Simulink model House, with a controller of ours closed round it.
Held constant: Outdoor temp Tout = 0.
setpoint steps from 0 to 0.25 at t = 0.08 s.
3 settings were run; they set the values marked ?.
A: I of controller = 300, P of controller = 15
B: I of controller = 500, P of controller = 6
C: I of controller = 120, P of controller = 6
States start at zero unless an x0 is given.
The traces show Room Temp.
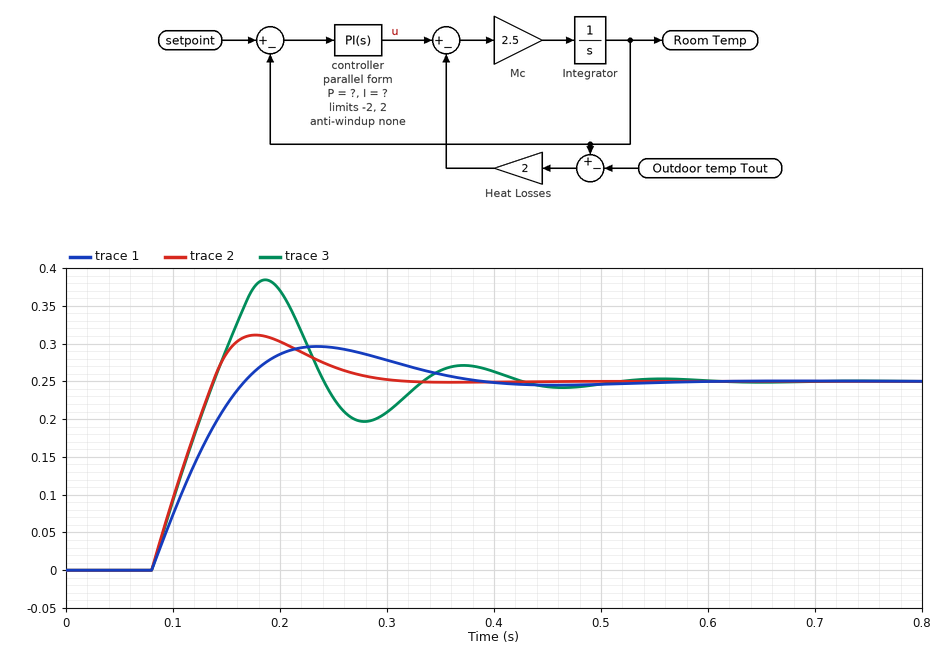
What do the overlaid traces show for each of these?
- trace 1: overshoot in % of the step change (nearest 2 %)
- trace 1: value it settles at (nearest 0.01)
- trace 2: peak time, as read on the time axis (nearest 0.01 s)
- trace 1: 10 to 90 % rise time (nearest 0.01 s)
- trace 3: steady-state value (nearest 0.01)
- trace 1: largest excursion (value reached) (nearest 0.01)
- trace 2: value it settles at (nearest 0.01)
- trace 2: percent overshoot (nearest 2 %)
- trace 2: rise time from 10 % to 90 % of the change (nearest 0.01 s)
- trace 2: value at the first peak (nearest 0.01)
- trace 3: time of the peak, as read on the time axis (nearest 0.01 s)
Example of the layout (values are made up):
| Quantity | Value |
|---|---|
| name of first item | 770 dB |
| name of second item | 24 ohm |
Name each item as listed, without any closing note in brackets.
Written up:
| Quantity | Value |
|---|---|
| trace 1: overshoot in % of the step change | 18 % |
| trace 1: value it settles at | 0.25 |
| trace 2: peak time, as read on the time axis | 0.18 s |
| trace 1: 10 to 90 % rise time | 0.07 s |
| trace 3: steady-state value | 0.25 |
| trace 1: largest excursion (value reached) | 0.30 |
| trace 2: value it settles at | 0.25 |
| trace 2: percent overshoot | 24 % |
| trace 2: rise time from 10 % to 90 % of the change | 0.05 s |
| trace 2: value at the first peak | 0.31 |
| trace 3: time of the peak, as read on the time axis | 0.19 s |
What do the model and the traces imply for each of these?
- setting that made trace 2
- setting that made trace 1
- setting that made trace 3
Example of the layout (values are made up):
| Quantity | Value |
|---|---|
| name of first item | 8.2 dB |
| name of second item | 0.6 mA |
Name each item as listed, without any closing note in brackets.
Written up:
| Quantity | Value |
|---|---|
| setting that made trace 2 | A |
| setting that made trace 1 | C |
| setting that made trace 3 | B |
